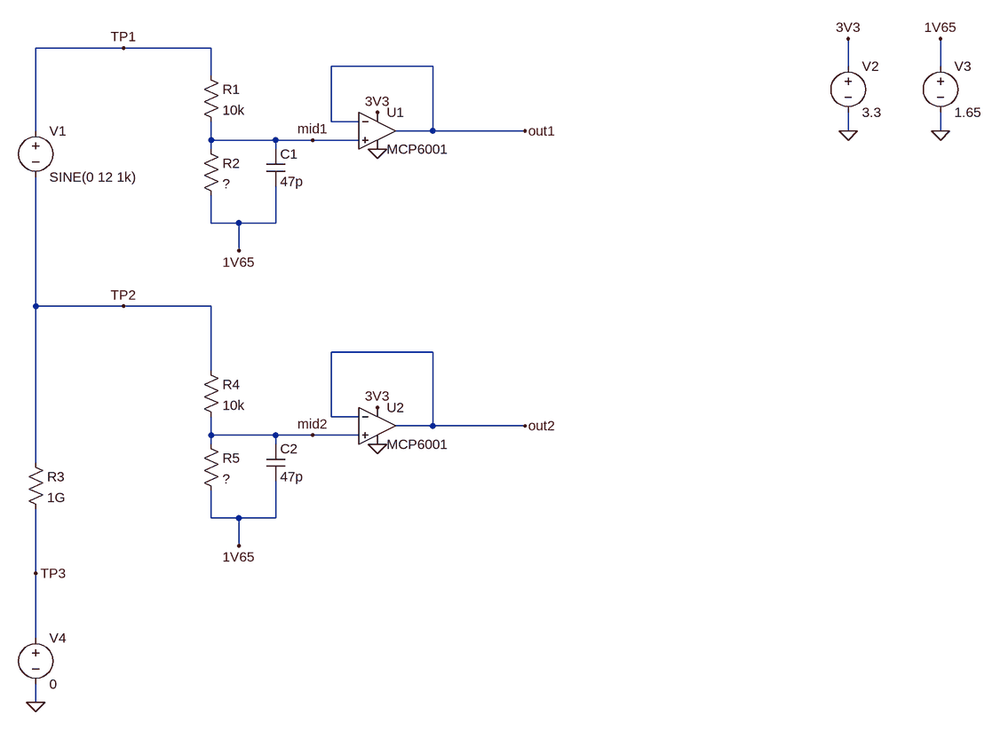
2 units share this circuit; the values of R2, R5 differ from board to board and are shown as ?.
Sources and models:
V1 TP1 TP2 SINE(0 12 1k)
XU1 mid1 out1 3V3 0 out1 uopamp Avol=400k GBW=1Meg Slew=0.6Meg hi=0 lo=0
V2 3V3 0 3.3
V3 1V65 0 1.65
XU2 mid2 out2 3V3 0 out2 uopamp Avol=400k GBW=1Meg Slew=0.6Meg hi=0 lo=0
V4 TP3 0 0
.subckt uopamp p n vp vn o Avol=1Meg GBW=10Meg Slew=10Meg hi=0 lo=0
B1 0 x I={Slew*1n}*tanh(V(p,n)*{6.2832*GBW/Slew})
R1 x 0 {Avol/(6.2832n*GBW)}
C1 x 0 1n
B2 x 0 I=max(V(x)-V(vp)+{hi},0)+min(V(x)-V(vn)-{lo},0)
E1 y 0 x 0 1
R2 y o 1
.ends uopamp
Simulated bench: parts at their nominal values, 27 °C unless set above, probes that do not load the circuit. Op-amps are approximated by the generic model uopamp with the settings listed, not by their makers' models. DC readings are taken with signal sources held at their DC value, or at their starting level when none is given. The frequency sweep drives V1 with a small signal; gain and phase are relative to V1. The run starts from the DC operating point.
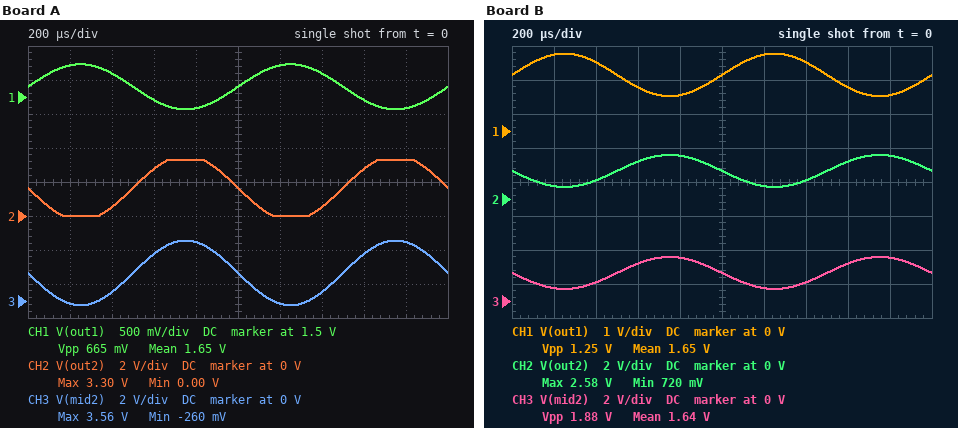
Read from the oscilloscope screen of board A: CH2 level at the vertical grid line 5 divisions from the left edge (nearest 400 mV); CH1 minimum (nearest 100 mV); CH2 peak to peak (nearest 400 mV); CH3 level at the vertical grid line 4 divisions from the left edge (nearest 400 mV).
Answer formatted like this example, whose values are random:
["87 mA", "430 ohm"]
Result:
["1.6 V", "1.3 V", "3.2 V", "3.6 V"]
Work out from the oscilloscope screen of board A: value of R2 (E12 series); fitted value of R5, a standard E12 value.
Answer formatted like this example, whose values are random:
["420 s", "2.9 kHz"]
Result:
["680 Ω", "3.9 kΩ"]
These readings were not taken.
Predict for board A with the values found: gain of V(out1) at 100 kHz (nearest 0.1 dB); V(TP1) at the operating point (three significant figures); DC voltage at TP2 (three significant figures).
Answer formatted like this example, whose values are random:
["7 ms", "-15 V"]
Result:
["-31.2 dB", "1.65 V", "1.65 V"]
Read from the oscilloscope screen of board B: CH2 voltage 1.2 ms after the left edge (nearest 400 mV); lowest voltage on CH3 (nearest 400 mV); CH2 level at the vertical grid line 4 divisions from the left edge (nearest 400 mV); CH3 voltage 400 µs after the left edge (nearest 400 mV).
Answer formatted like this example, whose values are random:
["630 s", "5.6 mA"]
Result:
["800 mV", "800 mV", "2.4 V", "1.2 V"]
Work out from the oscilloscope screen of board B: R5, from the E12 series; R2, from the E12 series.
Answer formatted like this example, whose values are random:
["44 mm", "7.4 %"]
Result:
["1.8 kΩ", "1.2 kΩ"]
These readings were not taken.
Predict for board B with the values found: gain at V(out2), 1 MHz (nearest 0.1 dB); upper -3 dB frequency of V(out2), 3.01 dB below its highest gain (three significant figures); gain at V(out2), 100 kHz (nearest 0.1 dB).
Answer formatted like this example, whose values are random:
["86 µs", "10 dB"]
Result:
["-26.0 dB", "848 kHz", "-22.2 dB"]
